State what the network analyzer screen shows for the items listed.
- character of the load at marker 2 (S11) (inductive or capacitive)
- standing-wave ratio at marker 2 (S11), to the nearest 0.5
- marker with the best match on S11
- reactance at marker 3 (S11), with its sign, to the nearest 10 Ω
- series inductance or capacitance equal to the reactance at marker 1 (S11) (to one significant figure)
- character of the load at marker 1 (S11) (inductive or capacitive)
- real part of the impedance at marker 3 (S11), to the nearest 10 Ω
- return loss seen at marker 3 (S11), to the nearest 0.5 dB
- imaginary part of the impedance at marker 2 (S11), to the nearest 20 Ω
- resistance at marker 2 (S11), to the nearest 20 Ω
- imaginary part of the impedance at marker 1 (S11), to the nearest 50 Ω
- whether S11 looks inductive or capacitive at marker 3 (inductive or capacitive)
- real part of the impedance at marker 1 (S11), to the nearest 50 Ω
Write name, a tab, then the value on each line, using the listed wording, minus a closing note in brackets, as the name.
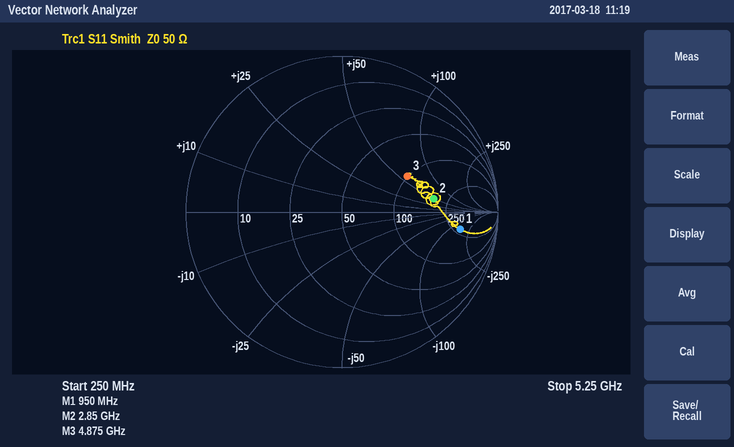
character of the load at marker 2 (S11)	inductive
standing-wave ratio at marker 2 (S11), to the nearest 0.5	4.0
marker with the best match on S11	marker 3
reactance at marker 3 (S11), with its sign, to the nearest 10 Ω	+60 Ω
series inductance or capacitance equal to the reactance at marker 1 (S11)	1 pF
character of the load at marker 1 (S11)	capacitive
real part of the impedance at marker 3 (S11), to the nearest 10 Ω	100 Ω
return loss seen at marker 3 (S11), to the nearest 0.5 dB	6.5 dB
imaginary part of the impedance at marker 2 (S11), to the nearest 20 Ω	+40 Ω
resistance at marker 2 (S11), to the nearest 20 Ω	180 Ω
imaginary part of the impedance at marker 1 (S11), to the nearest 50 Ω	-150 Ω
whether S11 looks inductive or capacitive at marker 3	inductive
real part of the impedance at marker 1 (S11), to the nearest 50 Ω	300 Ω
